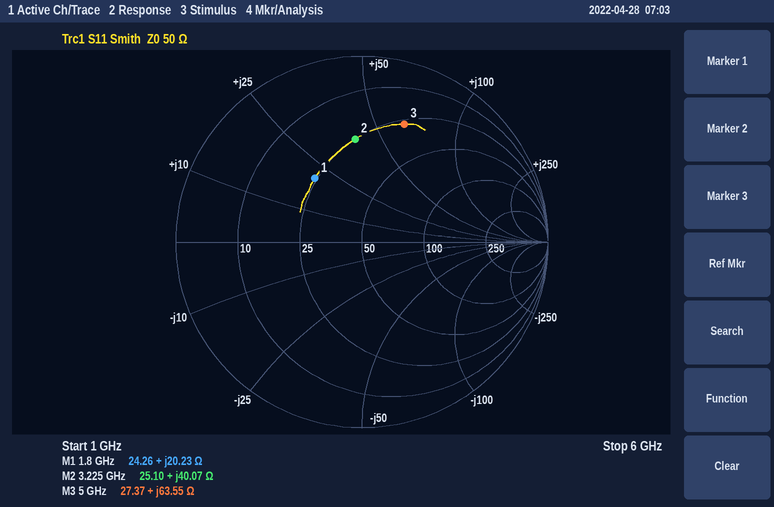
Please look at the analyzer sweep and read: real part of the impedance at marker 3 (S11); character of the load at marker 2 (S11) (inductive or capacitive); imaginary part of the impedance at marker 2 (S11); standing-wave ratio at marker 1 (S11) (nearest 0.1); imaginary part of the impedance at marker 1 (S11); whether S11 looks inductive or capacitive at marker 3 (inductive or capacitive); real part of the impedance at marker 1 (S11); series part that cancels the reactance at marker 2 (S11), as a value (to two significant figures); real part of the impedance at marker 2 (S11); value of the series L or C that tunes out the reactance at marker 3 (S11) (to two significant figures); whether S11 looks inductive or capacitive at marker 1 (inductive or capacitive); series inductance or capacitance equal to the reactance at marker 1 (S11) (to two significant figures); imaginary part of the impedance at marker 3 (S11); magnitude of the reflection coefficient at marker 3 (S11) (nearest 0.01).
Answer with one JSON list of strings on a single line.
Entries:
["27.37 Ω", "inductive", "+40.07 Ω", "2.5", "+20.23 Ω", "inductive", "24.26 Ω", "1.2 pF", "25.10 Ω", "500 fF", "inductive", "1.8 nH", "+63.55 Ω", "0.67"]
